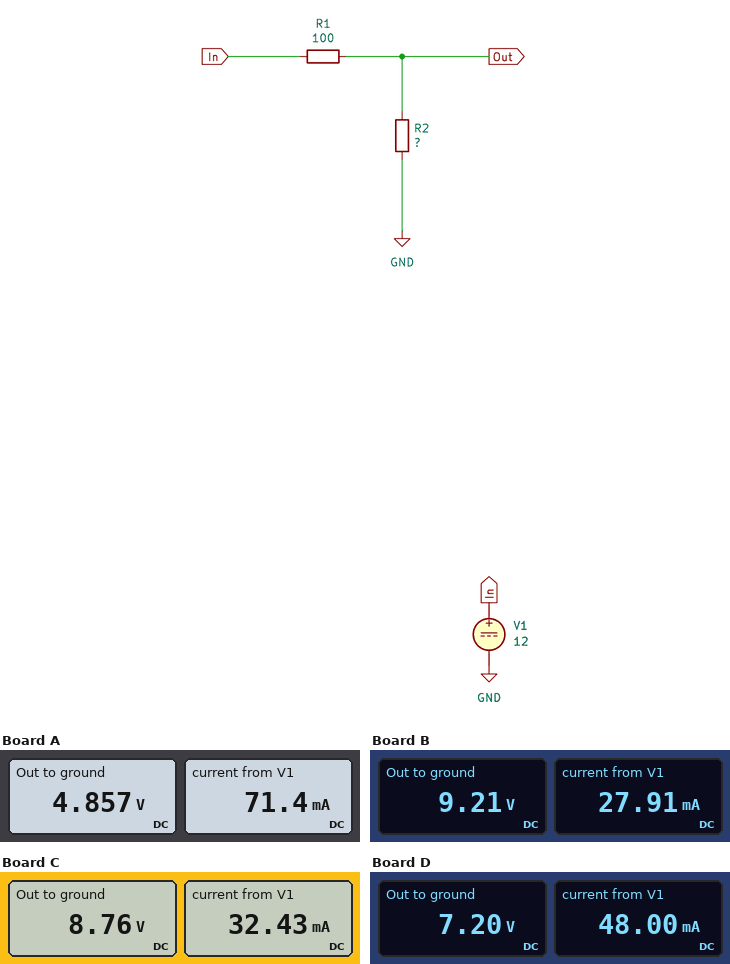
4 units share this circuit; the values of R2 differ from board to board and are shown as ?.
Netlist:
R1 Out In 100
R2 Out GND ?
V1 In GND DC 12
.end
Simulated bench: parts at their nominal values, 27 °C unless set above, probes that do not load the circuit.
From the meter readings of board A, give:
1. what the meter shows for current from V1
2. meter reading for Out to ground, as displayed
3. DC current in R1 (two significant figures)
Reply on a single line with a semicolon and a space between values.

71.4 mA; 4.857 V; 71 mA
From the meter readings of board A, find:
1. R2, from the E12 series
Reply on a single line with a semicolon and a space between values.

68 Ω
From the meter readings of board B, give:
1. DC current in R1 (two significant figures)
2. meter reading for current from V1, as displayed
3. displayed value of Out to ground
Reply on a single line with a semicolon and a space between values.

28 mA; 27.91 mA; 9.21 V
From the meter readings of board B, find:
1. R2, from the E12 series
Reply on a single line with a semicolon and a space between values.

330 Ω
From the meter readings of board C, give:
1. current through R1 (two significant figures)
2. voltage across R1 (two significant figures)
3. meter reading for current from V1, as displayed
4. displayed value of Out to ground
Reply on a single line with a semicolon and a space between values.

32 mA; 3.2 V; 32.43 mA; 8.76 V
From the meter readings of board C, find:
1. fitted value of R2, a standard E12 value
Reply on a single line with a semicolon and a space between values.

270 Ω
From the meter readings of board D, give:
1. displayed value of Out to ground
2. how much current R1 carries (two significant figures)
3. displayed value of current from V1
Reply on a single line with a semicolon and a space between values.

7.20 V; 48 mA; 48.00 mA
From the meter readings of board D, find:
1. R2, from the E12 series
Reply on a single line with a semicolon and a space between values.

150 Ω
